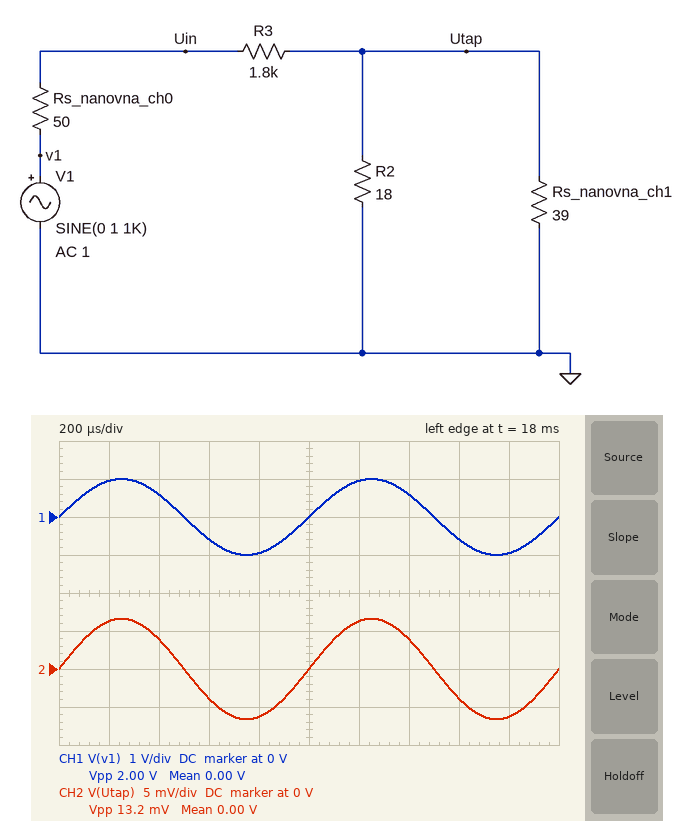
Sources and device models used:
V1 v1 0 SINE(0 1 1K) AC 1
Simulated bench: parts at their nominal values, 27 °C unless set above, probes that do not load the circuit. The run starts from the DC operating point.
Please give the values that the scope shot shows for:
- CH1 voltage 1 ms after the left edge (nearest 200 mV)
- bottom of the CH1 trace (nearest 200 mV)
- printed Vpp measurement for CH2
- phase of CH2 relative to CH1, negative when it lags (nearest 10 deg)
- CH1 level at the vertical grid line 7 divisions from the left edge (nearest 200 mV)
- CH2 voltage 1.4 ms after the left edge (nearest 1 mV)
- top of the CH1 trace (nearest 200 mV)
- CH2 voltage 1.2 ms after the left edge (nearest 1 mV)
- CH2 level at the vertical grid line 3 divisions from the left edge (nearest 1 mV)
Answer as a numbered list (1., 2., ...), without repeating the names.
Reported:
1. 0 V
2. -1.0 V
3. 13.2 mV
4. 0 deg
5. 600 mV
6. 4 mV
7. 1.0 V
8. 6 mV
9. -4 mV
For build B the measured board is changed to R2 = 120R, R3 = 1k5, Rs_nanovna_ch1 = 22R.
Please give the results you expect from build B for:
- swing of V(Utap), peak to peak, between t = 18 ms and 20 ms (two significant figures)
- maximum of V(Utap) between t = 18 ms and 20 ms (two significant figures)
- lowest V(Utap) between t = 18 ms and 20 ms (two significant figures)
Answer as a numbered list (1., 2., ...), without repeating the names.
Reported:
1. 24 mV
2. 12 mV
3. -12 mV
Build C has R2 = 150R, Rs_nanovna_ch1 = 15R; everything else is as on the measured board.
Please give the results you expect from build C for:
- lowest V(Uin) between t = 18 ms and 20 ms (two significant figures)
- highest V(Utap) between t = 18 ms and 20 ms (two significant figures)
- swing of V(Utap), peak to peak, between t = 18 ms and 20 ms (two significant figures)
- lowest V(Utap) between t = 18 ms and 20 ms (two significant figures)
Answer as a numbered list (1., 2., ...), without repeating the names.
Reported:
1. -970 mV
2. 7.3 mV
3. 15 mV
4. -7.3 mV
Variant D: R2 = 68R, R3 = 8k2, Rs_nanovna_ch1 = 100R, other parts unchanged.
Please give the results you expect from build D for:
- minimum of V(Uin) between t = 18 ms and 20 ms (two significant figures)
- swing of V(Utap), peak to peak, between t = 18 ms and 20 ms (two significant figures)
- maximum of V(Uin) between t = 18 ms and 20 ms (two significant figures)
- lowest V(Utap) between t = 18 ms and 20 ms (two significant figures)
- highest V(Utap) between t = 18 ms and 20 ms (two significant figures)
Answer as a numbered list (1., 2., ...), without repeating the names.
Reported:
1. -990 mV
2. 9.8 mV
3. 990 mV
4. -4.9 mV
5. 4.9 mV
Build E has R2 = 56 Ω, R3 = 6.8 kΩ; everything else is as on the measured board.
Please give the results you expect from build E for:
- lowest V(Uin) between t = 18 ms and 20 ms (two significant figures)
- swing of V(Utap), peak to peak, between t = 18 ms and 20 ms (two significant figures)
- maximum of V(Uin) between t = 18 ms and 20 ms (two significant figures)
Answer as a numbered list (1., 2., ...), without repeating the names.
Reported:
1. -990 mV
2. 6.7 mV
3. 990 mV
